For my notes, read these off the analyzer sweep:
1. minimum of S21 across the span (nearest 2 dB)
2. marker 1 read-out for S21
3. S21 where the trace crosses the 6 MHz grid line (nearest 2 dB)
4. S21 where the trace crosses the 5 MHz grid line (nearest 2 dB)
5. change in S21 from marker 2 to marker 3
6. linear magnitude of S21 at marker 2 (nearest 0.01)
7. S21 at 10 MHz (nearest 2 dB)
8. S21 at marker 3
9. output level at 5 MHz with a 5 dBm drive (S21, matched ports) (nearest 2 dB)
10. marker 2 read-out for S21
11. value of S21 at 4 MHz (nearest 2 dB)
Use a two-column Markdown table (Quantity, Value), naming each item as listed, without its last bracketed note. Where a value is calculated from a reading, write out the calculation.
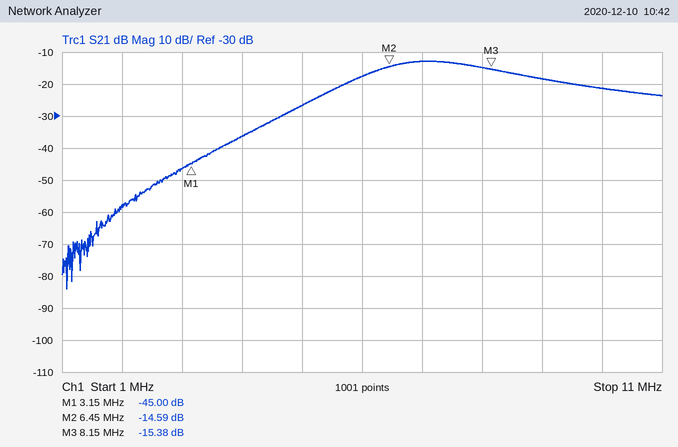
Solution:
| Quantity | Value |
|---|---|
| minimum of S21 across the span | -84 dB |
| marker 1 read-out for S21 | -45.00 dB |
| S21 where the trace crosses the 6 MHz grid line | -18 dB |
| S21 where the trace crosses the 5 MHz grid line | -26 dB |
| change in S21 from marker 2 to marker 3 | -15.38 − (-14.59) = -0.79 dB |
| linear magnitude of S21 at marker 2 | 10^(-14.59/20) ≈ 0.19 |
| S21 at 10 MHz | -22 dB |
| S21 at marker 3 | -15.38 dB |
| output level at 5 MHz with a 5 dBm drive (S21, matched ports) | 5 dBm + (-26 dB) = -22 dBm |
| marker 2 read-out for S21 | -14.59 dB |
| value of S21 at 4 MHz | -36 dB |
